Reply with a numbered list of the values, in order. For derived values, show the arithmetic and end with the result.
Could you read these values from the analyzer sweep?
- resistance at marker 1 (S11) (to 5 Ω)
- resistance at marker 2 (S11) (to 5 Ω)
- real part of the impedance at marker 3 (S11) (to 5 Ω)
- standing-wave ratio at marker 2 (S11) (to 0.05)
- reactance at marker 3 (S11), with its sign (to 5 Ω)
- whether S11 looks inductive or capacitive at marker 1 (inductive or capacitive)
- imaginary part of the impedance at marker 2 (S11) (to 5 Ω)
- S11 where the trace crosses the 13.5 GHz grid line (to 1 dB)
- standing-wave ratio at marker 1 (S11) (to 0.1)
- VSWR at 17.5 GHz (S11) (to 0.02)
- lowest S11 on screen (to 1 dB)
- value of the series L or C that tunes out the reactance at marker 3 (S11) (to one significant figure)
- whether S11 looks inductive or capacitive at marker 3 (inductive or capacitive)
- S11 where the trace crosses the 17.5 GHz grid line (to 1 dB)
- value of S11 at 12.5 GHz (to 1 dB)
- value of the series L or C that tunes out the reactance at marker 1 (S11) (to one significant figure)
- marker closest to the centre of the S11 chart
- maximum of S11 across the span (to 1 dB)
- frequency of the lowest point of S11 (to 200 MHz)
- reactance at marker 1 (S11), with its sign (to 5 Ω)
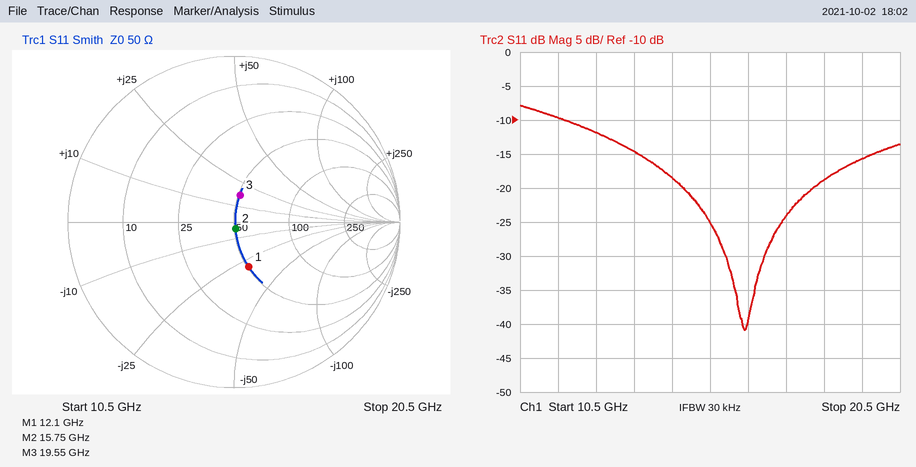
1. 50 Ω
2. 50 Ω
3. 50 Ω
4. 1.10
5. +15 Ω
6. capacitive
7. -5 Ω
8. -15 dB
9. 1.8
10. |Γ| = 10^(-24/20) = 0.0631; VSWR = (1 + 0.0631)/(1 − 0.0631) ≈ 1.13, so 1.14 to the nearest 0.02
11. -41 dB
12. C = 1/(2π × 19.55 GHz × 15 Ω) ≈ 543 fF, so 500 fF to one significant figure
13. inductive
14. -24 dB
15. -12 dB
16. L = 30 Ω/(2π × 12.1 GHz) ≈ 395 pH, so 400 pH to one significant figure
17. marker 2
18. -8 dB
19. 16.4 GHz
20. -30 Ω
